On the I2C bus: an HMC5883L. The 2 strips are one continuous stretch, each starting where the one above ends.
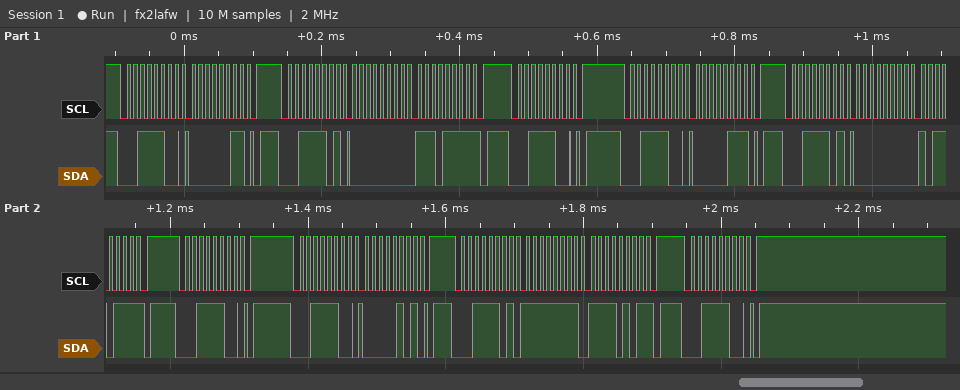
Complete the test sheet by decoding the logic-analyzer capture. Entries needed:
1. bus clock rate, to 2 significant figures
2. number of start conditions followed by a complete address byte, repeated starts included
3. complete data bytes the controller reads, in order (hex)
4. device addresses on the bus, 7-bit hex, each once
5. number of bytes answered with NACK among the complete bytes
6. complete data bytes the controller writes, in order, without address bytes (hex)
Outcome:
100 kHz
9
00 EF 00 B7 FF F5
0x1E
3
03 07 05
